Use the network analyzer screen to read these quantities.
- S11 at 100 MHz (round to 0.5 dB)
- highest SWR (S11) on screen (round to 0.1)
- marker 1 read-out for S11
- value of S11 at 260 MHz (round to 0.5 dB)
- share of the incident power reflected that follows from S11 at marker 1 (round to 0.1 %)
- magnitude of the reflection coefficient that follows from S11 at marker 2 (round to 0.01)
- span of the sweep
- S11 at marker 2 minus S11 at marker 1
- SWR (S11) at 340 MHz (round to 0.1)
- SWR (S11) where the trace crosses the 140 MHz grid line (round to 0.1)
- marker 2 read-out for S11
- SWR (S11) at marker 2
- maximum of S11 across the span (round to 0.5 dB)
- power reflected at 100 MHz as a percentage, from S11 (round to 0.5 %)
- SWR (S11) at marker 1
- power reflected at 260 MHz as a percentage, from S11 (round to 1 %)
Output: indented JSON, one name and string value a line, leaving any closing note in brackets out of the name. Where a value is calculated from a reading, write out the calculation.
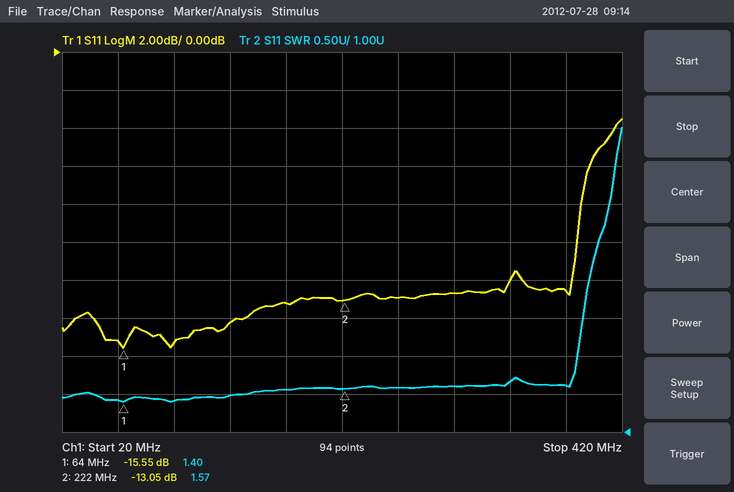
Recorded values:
{
  "S11 at 100 MHz": "-15.5 dB",
  "highest SWR (S11) on screen": "5.0",
  "marker 1 read-out for S11": "-15.55 dB",
  "value of S11 at 260 MHz": "-13.0 dB",
  "share of the incident power reflected that follows from S11 at marker 1": "10^(-15.55/10) ≈ 2.8 %",
  "magnitude of the reflection coefficient that follows from S11 at marker 2": "10^(-13.05/20) ≈ 0.22",
  "span of the sweep": "400 MHz",
  "S11 at marker 2 minus S11 at marker 1": "-13.05 − (-15.55) = 2.50 dB",
  "SWR (S11) at 340 MHz": "1.7",
  "SWR (S11) where the trace crosses the 140 MHz grid line": "1.5",
  "marker 2 read-out for S11": "-13.05 dB",
  "SWR (S11) at marker 2": "1.57",
  "maximum of S11 across the span": "-3.5 dB",
  "power reflected at 100 MHz as a percentage, from S11": "10^(-15.5/10) ≈ 2.82 %, so 3.0 % to the nearest 0.5 %",
  "SWR (S11) at marker 1": "1.40",
  "power reflected at 260 MHz as a percentage, from S11": "10^(-13/10) ≈ 5 %"
}
